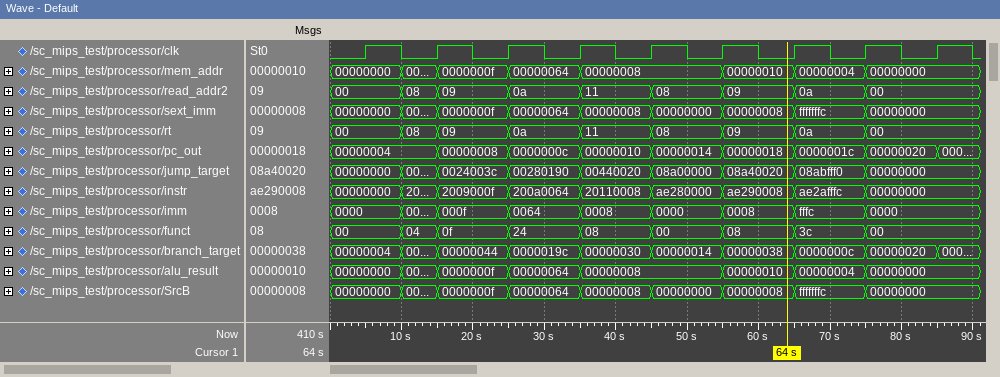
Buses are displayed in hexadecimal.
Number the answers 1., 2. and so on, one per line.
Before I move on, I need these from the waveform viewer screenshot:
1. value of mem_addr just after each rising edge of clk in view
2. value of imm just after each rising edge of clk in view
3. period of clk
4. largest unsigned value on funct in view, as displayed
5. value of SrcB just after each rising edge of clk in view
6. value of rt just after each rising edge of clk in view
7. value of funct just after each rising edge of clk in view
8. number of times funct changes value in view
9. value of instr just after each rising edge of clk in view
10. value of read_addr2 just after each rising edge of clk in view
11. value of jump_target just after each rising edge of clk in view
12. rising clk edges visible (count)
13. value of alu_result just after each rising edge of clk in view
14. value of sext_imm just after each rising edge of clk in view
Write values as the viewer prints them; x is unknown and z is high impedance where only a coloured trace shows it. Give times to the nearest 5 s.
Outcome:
1. 00000000, 0000000f, 00000064, 00000008, 00000008, 00000010, 00000004, 00000000, 00000000
2. 0000, 000f, 0064, 0008, 0000, 0008, fffc, 0000, 0000
3. 10 s
4. 3c
5. 00000000, 0000000f, 00000064, 00000008, 00000000, 00000008, fffffffc, 00000000, 00000000
6. 00, 09, 0a, 11, 08, 09, 0a, 00, 00
7. 00, 0f, 24, 08, 00, 08, 3c, 00, 00
8. 8
9. 00000000, 2009000f, 200a0064, 20110008, ae280000, ae290008, ae2afffc, 00000000, 00000000
10. 00, 09, 0a, 11, 08, 09, 0a, 00, 00
11. 00000000, 0024003c, 00280190, 00440020, 08a00000, 08a40020, 08abfff0, 00000000, 00000000
12. 9
13. 00000000, 0000000f, 00000064, 00000008, 00000008, 00000010, 00000004, 00000000, 00000000
14. 00000000, 0000000f, 00000064, 00000008, 00000000, 00000008, fffffffc, 00000000, 00000000
